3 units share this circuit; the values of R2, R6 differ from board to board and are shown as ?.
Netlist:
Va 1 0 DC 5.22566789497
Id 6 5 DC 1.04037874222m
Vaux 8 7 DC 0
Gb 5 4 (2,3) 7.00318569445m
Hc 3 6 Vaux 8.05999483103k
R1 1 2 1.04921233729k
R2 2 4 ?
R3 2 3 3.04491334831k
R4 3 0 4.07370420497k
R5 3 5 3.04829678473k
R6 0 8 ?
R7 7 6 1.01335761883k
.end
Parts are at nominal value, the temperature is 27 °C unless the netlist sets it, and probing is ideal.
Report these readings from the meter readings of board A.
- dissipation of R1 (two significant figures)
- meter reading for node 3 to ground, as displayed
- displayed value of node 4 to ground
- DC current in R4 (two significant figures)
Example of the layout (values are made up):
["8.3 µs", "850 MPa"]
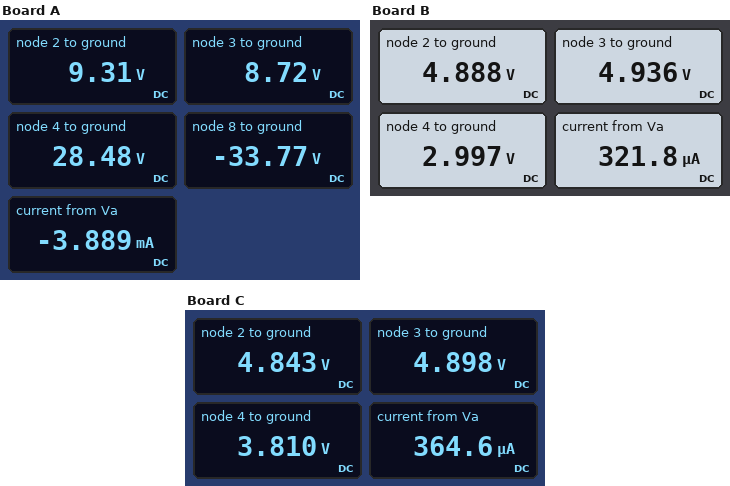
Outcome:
["16 mW", "8.72 V", "28.48 V", "2.1 mA"]
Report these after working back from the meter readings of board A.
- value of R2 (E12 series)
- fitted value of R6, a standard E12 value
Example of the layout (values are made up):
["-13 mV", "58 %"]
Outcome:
["4.7 kΩ", "5.6 kΩ"]
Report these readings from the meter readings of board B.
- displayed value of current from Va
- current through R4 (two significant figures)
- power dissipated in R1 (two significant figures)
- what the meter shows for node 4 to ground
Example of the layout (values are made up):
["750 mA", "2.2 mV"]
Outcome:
["321.8 µA", "1.2 mA", "110 µW", "2.997 V"]
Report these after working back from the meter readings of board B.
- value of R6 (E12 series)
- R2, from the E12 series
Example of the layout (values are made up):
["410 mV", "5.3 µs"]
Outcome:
["1.5 kΩ", "5.6 kΩ"]
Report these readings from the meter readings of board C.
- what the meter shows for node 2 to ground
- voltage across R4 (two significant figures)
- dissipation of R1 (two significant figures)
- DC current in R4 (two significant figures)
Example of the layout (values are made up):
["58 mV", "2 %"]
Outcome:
["4.843 V", "4.9 V", "140 µW", "1.2 mA"]
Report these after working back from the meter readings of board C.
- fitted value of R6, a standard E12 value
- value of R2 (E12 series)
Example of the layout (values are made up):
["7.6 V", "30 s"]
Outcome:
["1.2 kΩ", "2.7 kΩ"]
